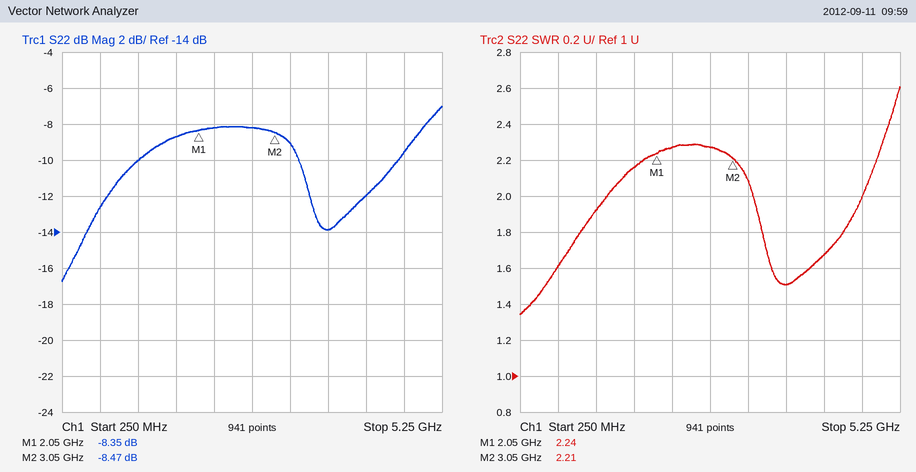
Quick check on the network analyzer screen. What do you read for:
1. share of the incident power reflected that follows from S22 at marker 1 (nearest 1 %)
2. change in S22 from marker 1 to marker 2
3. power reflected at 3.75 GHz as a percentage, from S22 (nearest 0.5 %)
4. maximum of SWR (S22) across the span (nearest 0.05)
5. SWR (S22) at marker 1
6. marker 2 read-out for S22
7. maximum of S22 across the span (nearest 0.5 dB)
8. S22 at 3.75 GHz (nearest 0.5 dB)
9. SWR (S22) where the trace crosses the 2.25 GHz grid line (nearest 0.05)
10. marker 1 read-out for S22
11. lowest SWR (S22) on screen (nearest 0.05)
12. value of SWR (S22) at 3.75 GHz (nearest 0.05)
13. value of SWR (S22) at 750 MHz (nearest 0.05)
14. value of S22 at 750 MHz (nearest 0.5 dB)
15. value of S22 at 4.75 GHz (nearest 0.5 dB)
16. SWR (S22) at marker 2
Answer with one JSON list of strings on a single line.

["15 %", "-0.12 dB", "4.0 %", "2.60", "2.24", "-8.47 dB", "-7.0 dB", "-14.0 dB", "2.25", "-8.35 dB", "1.35", "1.50", "1.60", "-12.5 dB", "-9.5 dB", "2.21"]
